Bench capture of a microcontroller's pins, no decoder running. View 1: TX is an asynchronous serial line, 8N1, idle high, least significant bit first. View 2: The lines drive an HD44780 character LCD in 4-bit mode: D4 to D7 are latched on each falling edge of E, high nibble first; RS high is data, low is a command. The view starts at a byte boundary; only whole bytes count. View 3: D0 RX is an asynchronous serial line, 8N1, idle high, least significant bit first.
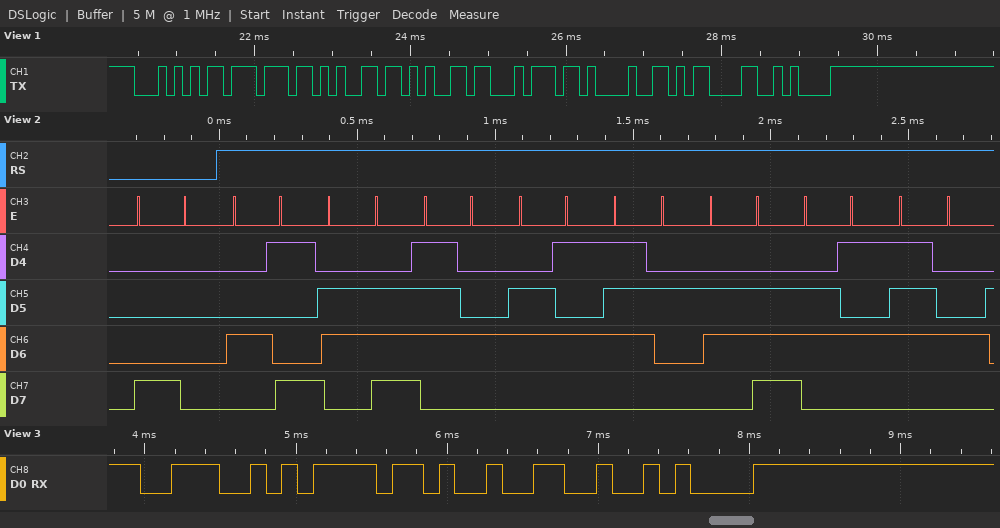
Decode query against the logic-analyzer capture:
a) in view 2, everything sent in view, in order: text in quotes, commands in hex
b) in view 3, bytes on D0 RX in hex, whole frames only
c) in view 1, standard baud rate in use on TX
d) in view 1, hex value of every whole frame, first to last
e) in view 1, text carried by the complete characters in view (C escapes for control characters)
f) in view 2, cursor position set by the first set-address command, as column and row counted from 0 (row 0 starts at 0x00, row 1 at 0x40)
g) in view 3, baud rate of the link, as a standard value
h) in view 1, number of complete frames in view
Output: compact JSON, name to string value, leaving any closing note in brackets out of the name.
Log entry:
{"in view 2, everything sent in view, in order: text in quotes, commands in hex": "0x80 \"Internet\"", "in view 3, bytes on D0 RX in hex, whole frames only": "4E 6F 32 0A", "in view 1, standard baud rate in use on TX": "9600 baud", "in view 1, hex value of every whole frame, first to last": "0x54 0x77 0x65 0x65 0x74 0x21 0x0D 0x0A", "in view 1, text carried by the complete characters in view": "\"Tweet!\\r\\n\"", "in view 2, cursor position set by the first set-address command, as column and row counted from 0": "column 0, row 0", "in view 3, baud rate of the link, as a standard value": "9600 baud", "in view 1, number of complete frames in view": "8"}
